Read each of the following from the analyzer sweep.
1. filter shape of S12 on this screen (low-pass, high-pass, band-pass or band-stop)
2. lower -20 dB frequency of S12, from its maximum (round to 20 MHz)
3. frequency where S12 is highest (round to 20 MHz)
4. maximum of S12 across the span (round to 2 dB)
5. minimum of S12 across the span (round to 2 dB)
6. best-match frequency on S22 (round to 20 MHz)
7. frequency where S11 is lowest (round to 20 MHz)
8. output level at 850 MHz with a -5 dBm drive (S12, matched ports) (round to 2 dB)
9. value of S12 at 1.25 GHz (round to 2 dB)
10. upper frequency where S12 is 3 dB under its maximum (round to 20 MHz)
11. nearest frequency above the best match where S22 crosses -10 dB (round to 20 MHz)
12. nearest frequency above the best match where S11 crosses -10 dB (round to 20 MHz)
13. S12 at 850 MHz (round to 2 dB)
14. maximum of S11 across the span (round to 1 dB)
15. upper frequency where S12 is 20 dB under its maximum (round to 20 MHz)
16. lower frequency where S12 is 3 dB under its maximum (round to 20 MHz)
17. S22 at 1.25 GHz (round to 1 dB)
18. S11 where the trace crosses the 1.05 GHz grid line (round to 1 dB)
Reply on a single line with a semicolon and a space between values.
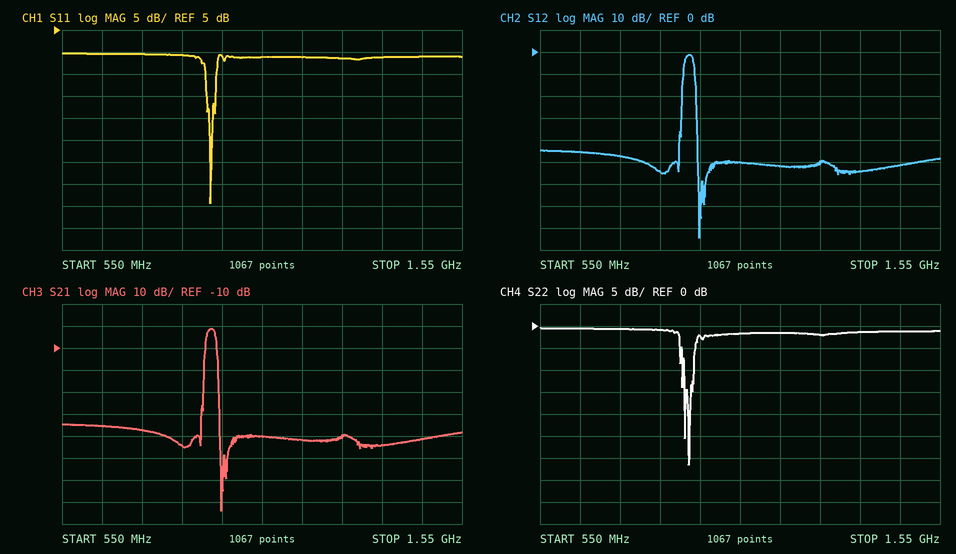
band-pass; 900 MHz; 920 MHz; -2 dB; -84 dB; 920 MHz; 920 MHz; -60 dBm; -50 dB; 940 MHz; 940 MHz; 940 MHz; -54 dB; 0 dB; 940 MHz; 920 MHz; -2 dB; -1 dB
